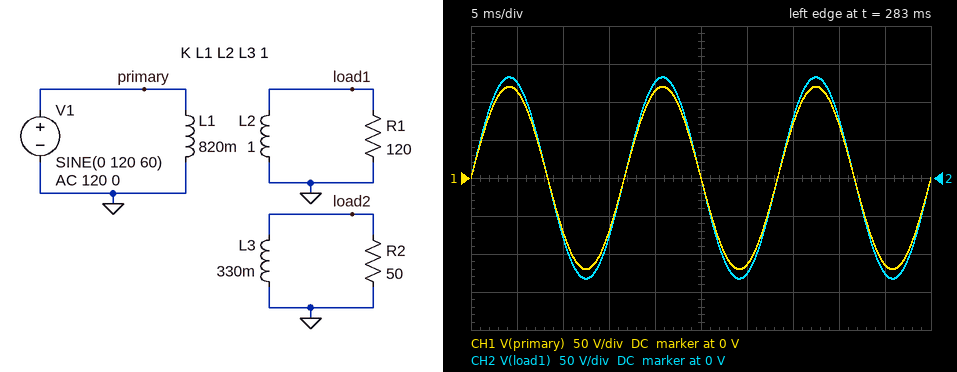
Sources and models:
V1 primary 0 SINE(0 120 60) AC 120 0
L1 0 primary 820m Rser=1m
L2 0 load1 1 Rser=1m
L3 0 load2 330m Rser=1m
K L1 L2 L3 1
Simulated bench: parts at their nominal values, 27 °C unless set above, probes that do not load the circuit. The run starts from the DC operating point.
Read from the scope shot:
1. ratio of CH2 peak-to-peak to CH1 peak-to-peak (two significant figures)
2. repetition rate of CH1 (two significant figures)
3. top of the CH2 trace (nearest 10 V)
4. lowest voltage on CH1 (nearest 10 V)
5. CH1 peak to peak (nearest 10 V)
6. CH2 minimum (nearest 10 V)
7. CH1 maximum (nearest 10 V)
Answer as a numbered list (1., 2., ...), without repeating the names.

1. 1.1
2. 60 Hz
3. 130 V
4. -120 V
5. 240 V
6. -130 V
7. 120 V
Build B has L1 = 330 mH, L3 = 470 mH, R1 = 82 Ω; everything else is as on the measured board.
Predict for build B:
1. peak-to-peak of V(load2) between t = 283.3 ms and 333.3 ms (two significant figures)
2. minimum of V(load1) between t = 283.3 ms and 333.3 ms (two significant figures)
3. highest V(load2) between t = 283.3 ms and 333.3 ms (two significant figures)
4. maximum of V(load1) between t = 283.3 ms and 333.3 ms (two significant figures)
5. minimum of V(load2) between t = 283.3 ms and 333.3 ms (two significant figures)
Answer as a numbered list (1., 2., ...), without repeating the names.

1. 290 V
2. -210 V
3. 140 V
4. 210 V
5. -140 V
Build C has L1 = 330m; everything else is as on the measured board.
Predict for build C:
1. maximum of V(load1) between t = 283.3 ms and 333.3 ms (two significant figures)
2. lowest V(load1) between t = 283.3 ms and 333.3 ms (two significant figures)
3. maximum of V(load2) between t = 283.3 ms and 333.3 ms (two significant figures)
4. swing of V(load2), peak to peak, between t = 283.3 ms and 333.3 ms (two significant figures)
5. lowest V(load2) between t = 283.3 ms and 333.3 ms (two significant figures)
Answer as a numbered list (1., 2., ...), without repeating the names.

1. 210 V
2. -210 V
3. 120 V
4. 240 V
5. -120 V
